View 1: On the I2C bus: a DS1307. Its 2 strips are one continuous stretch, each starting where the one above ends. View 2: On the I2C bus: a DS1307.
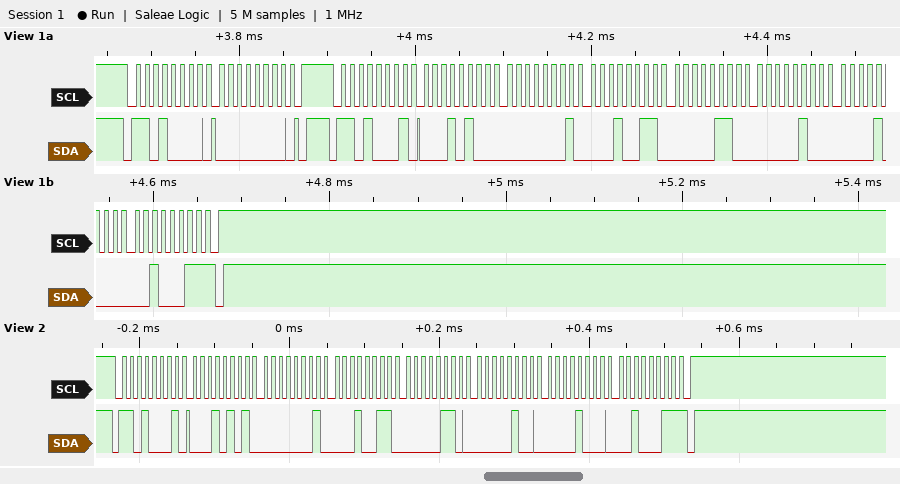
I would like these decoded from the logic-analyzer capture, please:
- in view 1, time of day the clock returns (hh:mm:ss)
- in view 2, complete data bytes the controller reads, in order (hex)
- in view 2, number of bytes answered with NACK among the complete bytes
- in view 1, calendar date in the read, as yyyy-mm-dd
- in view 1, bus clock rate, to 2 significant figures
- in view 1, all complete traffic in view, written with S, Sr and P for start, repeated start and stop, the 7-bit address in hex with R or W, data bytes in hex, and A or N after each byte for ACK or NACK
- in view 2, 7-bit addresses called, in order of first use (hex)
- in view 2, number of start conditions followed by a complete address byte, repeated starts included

13:01:14
15 01 13 06 04 08 23
1
2023-08-04
100 kHz
S 68W A 00 A P S 68R A 14 A 01 A 13 A 06 A 04 A 08 A 23 N P
0x68
1
